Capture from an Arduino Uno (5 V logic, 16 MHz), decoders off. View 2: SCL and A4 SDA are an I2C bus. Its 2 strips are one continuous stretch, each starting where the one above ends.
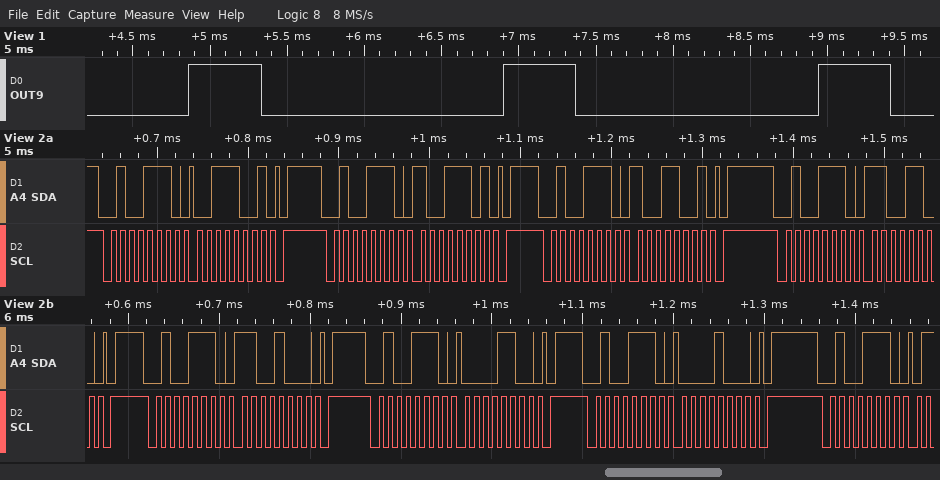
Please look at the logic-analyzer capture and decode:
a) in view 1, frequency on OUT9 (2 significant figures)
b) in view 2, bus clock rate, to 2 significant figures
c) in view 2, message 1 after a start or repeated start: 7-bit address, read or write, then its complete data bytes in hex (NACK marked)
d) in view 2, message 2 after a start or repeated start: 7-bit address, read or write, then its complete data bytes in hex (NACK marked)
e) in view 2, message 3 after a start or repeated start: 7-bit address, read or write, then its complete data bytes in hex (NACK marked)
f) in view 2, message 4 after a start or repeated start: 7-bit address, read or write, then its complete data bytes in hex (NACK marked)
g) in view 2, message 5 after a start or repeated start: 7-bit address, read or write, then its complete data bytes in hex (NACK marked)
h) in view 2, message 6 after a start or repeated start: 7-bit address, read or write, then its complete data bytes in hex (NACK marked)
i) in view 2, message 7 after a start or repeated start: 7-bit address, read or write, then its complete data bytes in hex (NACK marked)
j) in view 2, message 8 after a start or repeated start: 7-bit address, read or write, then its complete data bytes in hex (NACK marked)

490 Hz
100 kHz
0x27 write: 39
0x27 write: 9D
0x27 write: 99
0x27 write: CC
0x27 write: C8
0x27 write: 0C
0x27 write: 08
0x27 write
